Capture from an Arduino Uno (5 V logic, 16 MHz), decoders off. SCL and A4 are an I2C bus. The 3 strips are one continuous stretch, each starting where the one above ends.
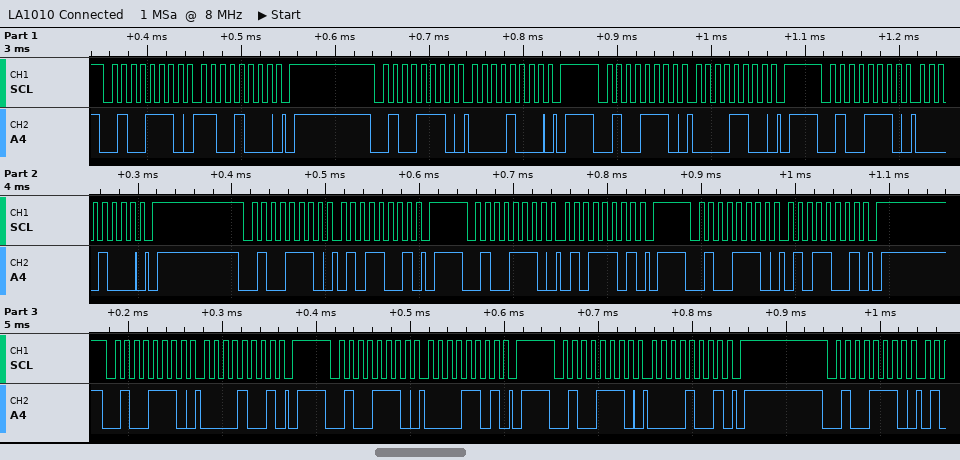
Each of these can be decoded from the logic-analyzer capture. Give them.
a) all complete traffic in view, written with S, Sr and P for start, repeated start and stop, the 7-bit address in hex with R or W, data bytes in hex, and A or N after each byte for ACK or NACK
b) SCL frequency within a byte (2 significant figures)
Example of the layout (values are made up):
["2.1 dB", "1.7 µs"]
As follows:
["S 27W A C8 A P S 27W A 08 A P S 27W A 0C A P S 27W A 08 A P S 27W A 59 A P S 27W A 5D A P S 27W A 59 A P S 27W A 09 A P S 27W A 0D A P S 27W A 09 A P S 27W A", "100 kHz"]
